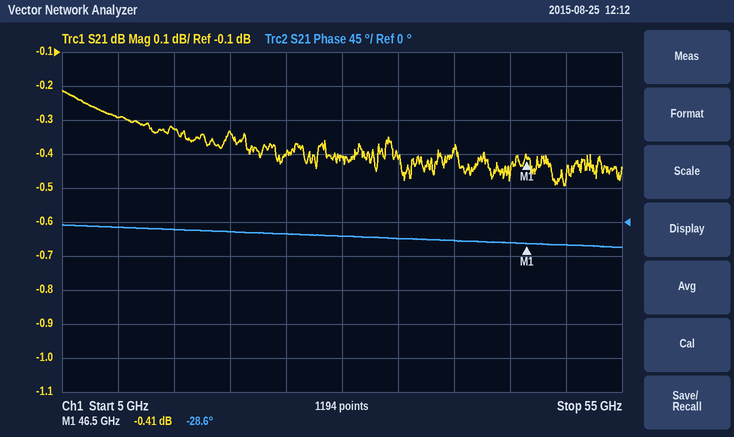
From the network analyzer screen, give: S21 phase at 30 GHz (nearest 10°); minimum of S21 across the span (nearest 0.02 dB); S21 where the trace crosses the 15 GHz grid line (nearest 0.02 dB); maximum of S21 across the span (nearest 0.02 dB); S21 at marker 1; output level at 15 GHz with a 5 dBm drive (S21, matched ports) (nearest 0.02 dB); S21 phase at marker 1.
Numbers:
-20°
-0.50 dB
-0.32 dB
-0.22 dB
-0.41 dB
4.68 dBm
-28.6°
